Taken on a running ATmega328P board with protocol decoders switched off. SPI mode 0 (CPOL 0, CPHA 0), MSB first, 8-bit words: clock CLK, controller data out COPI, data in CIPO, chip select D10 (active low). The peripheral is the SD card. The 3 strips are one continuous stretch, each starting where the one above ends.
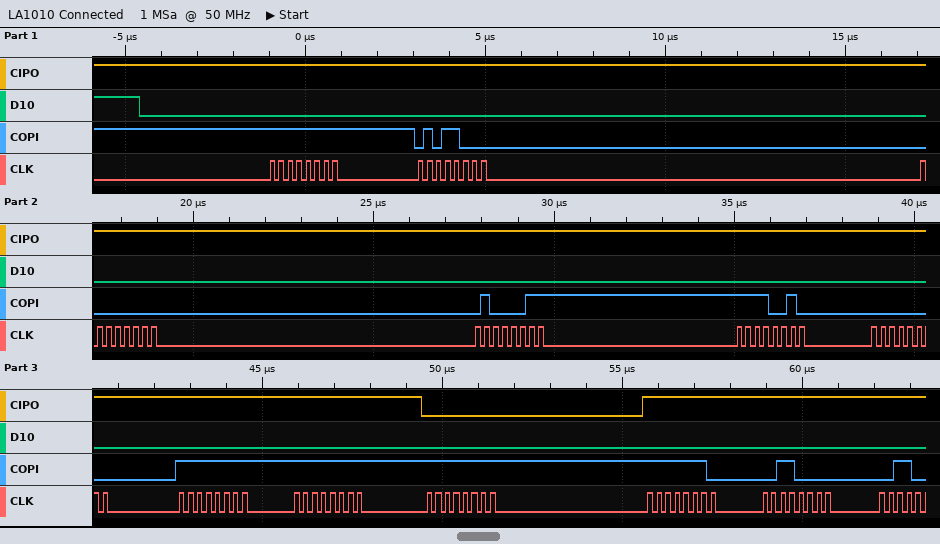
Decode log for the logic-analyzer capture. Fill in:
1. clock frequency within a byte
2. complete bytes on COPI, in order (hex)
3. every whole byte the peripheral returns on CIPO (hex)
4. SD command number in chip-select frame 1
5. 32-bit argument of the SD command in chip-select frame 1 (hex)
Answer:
4 MHz
FF 58 00 43 F2 00 FF FF FF FE 30
FF FF FF FF FF FF FF FF 00 FF FF
CMD24
0x0043F200
